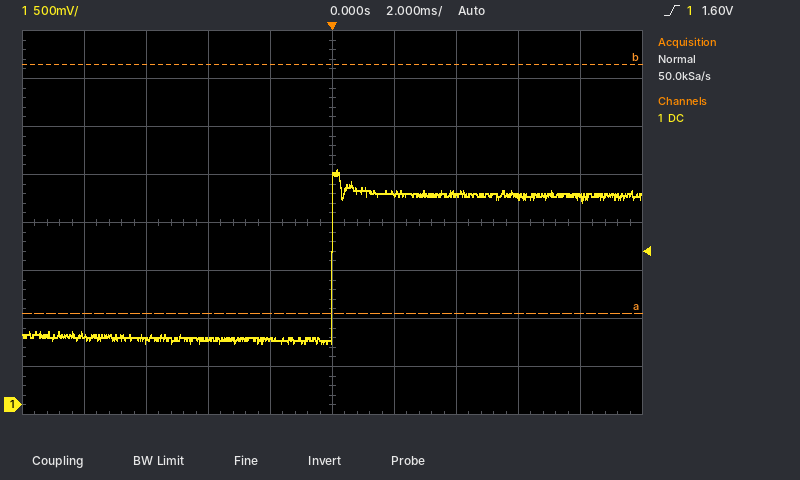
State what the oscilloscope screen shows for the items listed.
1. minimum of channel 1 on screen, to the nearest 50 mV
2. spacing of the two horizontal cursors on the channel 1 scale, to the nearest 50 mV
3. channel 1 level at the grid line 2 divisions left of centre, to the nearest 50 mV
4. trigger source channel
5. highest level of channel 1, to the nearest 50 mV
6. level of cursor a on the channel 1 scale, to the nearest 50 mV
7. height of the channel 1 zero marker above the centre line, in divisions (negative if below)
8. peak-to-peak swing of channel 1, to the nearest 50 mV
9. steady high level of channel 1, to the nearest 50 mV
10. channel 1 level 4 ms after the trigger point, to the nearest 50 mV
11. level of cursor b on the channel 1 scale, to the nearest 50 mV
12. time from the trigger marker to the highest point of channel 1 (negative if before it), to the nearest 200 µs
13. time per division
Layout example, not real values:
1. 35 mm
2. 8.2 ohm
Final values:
1. 650 mV
2. 2.60 V
3. 700 mV
4. channel 1
5. 2.45 V
6. 950 mV
7. -3.8 div
8. 1.80 V
9. 2.20 V
10. 2.20 V
11. 3.55 V
12. +200 µs
13. 2 ms
